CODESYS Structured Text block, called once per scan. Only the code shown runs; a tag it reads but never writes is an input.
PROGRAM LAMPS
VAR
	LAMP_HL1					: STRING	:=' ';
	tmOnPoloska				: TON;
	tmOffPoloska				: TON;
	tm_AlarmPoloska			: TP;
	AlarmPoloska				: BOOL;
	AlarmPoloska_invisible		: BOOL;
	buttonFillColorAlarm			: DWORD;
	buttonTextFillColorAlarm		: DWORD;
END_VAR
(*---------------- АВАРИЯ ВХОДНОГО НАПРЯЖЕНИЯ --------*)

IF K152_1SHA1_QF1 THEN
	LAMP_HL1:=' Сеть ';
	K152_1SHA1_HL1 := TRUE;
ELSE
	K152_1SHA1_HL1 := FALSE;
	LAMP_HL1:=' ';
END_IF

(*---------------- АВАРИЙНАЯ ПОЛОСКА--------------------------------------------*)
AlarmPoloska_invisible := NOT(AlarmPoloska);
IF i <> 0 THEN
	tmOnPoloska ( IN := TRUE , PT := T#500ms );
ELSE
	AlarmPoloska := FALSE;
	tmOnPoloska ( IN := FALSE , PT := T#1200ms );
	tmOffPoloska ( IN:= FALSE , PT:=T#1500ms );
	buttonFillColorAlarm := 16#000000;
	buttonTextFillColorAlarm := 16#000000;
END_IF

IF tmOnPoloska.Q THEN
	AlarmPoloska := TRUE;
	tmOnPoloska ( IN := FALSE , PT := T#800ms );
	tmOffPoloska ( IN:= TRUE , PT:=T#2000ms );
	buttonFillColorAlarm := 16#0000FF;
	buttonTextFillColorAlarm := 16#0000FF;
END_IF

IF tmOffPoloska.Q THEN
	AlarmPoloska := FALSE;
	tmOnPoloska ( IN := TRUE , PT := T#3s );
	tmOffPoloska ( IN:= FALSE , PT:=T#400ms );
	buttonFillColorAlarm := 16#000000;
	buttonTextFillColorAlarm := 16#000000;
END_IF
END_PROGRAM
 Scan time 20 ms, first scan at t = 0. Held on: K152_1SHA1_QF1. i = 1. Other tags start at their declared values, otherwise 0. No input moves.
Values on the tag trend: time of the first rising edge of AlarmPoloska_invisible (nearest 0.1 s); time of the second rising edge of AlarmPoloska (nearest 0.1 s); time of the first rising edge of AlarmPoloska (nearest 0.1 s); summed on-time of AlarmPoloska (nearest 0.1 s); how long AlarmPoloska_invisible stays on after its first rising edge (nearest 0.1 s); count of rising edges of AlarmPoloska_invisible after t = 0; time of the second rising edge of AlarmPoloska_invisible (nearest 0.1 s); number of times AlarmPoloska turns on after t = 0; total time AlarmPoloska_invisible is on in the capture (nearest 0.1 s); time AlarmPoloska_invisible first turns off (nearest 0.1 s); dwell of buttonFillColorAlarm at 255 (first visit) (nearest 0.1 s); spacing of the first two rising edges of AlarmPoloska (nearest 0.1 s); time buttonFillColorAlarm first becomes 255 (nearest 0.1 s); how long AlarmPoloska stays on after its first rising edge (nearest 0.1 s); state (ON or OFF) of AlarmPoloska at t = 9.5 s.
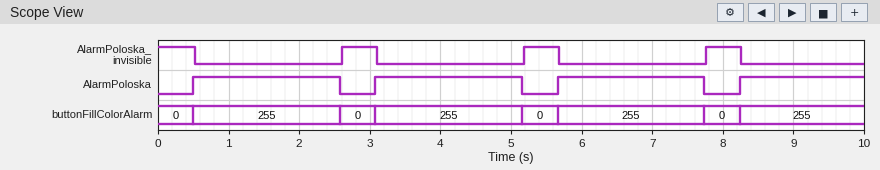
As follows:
2.6 s
3.1 s
0.5 s
8.0 s
0.5 s
3
5.2 s
4
2.0 s
0.5 s
2.1 s
2.6 s
0.5 s
2.1 s
ON
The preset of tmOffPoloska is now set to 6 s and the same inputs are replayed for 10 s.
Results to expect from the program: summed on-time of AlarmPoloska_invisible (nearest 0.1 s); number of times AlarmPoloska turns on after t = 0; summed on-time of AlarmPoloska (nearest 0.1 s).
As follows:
1.0 s
2
9.0 s
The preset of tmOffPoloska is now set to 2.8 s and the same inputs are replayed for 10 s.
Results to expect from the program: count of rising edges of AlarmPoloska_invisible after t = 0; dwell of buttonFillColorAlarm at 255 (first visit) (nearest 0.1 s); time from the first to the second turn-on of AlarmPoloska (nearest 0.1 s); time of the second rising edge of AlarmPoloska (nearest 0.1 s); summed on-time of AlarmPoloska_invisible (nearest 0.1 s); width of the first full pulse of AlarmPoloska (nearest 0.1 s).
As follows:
2
3.1 s
3.6 s
4.1 s
1.5 s
3.1 s
